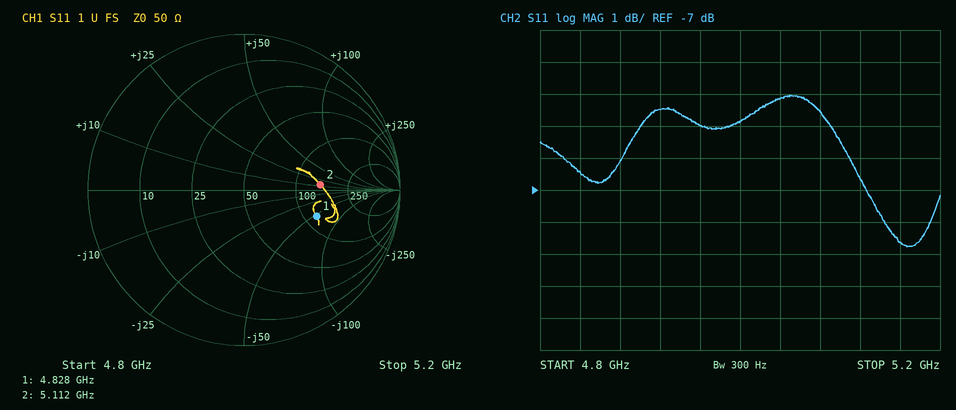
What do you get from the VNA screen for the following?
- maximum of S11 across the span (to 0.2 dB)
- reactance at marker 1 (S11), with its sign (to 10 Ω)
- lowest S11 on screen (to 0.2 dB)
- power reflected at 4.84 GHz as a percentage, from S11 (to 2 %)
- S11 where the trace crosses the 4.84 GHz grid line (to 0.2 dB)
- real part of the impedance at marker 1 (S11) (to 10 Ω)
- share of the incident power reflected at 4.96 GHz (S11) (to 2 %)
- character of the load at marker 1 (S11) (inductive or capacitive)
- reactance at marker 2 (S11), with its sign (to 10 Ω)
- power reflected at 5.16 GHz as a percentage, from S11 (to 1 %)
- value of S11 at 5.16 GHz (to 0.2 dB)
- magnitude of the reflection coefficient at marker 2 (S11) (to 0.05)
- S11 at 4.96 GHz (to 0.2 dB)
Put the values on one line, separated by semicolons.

-4.0 dB; -50 Ω; -8.8 dB; 22 %; -6.4 dB; 120 Ω; 32 %; capacitive; +10 Ω; 14 %; -8.6 dB; 0.50; -5.0 dB
